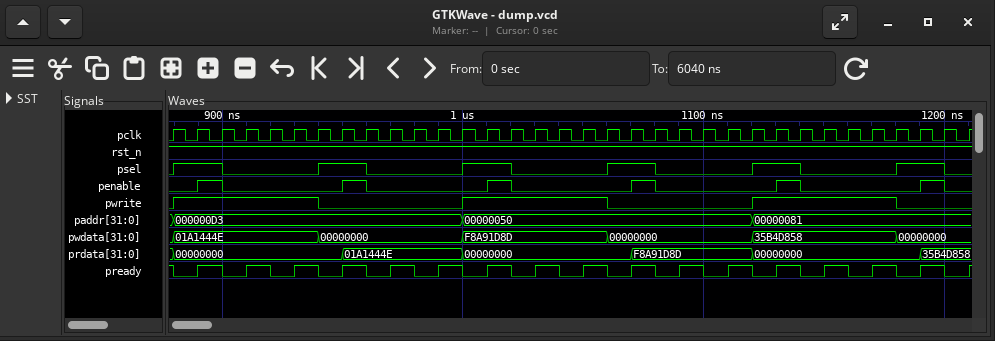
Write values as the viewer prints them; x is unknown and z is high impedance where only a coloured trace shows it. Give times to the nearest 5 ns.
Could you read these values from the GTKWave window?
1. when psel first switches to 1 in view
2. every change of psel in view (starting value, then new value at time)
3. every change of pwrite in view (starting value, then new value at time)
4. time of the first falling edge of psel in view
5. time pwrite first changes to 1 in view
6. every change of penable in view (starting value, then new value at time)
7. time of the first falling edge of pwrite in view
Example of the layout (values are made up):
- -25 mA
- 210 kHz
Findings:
- 880 ns
- 0, 1 at 880 ns, 0 at 900 ns, 1 at 940 ns, 0 at 960 ns, 1 at 1000 ns, 0 at 1020 ns, 1 at 1060 ns, 0 at 1080 ns, 1 at 1120 ns, 0 at 1140 ns, 1 at 1180 ns, 0 at 1200 ns
- 0, 1 at 880 ns, 0 at 940 ns, 1 at 1000 ns, 0 at 1060 ns, 1 at 1120 ns, 0 at 1180 ns
- 900 ns
- 880 ns
- 0, 1 at 890 ns, 0 at 900 ns, 1 at 950 ns, 0 at 960 ns, 1 at 1010 ns, 0 at 1020 ns, 1 at 1070 ns, 0 at 1080 ns, 1 at 1130 ns, 0 at 1140 ns, 1 at 1190 ns, 0 at 1200 ns
- 940 ns
